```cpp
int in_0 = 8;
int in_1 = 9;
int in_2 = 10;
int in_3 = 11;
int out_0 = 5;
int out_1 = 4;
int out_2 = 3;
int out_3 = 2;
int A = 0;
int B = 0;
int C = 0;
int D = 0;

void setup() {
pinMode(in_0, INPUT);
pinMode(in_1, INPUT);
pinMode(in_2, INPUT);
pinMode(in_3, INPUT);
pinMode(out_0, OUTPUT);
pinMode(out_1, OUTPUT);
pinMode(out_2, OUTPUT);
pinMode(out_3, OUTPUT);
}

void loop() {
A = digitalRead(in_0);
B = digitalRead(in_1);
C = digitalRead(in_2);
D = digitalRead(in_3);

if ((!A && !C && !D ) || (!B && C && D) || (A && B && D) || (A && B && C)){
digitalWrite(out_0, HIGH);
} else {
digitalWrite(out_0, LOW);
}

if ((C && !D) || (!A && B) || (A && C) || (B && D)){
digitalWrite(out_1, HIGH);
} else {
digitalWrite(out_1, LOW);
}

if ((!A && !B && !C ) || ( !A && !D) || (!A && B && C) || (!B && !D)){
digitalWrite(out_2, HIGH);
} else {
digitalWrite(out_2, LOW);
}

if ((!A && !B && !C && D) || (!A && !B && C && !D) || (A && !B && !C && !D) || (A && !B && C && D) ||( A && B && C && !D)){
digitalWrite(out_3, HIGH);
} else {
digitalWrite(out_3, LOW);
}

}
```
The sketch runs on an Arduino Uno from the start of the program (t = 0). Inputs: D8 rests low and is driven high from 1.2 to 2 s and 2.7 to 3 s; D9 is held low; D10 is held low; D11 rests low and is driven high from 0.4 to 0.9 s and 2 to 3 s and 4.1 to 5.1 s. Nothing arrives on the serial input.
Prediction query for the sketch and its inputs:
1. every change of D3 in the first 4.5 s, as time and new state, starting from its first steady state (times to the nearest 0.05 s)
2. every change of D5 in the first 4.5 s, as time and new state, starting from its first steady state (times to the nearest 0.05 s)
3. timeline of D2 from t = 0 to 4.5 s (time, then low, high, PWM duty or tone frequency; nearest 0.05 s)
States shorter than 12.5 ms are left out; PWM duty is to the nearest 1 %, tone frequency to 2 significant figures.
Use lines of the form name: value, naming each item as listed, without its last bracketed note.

every change of D3 in the first 4.5 s, as time and new state, starting from its first steady state: 0 s high; 2.7 s low; 3 s high
every change of D5 in the first 4.5 s, as time and new state, starting from its first steady state: 0 s high; 0.4 s low; 0.9 s high; 1.2 s low; 3 s high; 4.1 s low
timeline of D2 from t = 0 to 4.5 s: 0 s low; 0.4 s high; 0.9 s low; 1.2 s high; 2.7 s low; 4.1 s high
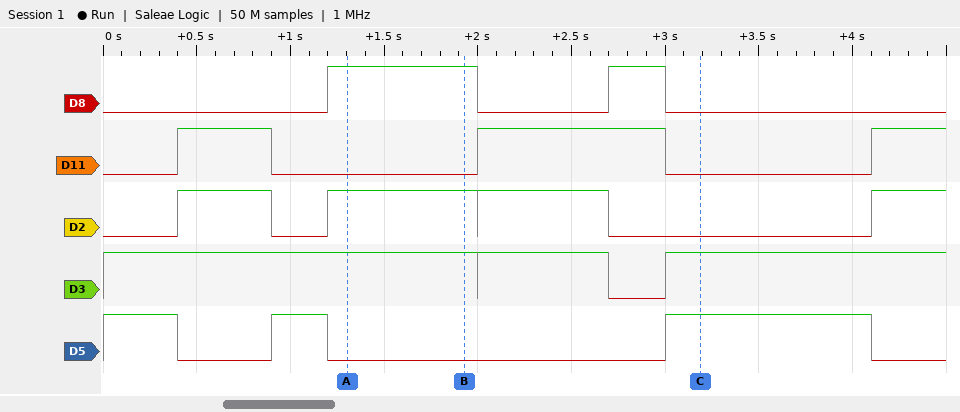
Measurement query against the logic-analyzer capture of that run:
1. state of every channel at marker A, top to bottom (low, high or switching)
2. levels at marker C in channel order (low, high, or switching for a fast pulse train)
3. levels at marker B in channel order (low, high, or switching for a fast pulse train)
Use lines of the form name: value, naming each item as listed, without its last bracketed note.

state of every channel at marker A, top to bottom: D8 high, D11 low, D2 high, D3 high, D5 low
levels at marker C in channel order: D8 low, D11 low, D2 low, D3 high, D5 high
levels at marker B in channel order: D8 high, D11 low, D2 high, D3 high, D5 low
